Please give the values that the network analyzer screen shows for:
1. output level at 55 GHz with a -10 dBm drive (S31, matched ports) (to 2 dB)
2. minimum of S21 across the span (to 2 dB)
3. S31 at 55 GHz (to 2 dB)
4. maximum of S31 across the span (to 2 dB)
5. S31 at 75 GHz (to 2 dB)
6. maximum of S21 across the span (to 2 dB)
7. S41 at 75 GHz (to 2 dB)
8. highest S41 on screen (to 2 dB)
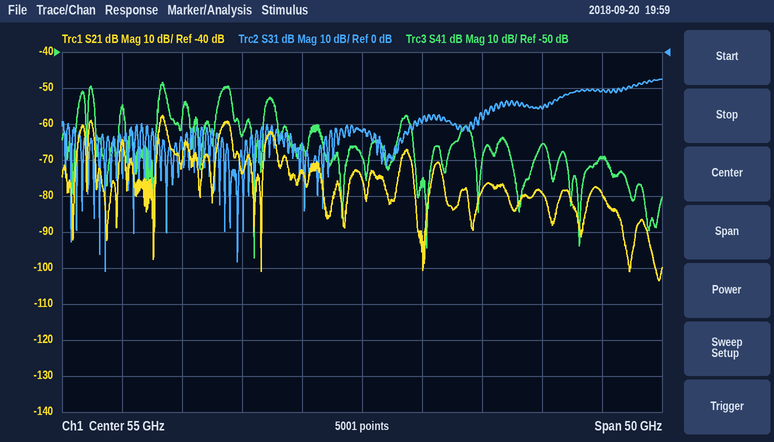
-32 dBm
-104 dB
-22 dB
-8 dB
-10 dB
-58 dB
-80 dB
-58 dB
